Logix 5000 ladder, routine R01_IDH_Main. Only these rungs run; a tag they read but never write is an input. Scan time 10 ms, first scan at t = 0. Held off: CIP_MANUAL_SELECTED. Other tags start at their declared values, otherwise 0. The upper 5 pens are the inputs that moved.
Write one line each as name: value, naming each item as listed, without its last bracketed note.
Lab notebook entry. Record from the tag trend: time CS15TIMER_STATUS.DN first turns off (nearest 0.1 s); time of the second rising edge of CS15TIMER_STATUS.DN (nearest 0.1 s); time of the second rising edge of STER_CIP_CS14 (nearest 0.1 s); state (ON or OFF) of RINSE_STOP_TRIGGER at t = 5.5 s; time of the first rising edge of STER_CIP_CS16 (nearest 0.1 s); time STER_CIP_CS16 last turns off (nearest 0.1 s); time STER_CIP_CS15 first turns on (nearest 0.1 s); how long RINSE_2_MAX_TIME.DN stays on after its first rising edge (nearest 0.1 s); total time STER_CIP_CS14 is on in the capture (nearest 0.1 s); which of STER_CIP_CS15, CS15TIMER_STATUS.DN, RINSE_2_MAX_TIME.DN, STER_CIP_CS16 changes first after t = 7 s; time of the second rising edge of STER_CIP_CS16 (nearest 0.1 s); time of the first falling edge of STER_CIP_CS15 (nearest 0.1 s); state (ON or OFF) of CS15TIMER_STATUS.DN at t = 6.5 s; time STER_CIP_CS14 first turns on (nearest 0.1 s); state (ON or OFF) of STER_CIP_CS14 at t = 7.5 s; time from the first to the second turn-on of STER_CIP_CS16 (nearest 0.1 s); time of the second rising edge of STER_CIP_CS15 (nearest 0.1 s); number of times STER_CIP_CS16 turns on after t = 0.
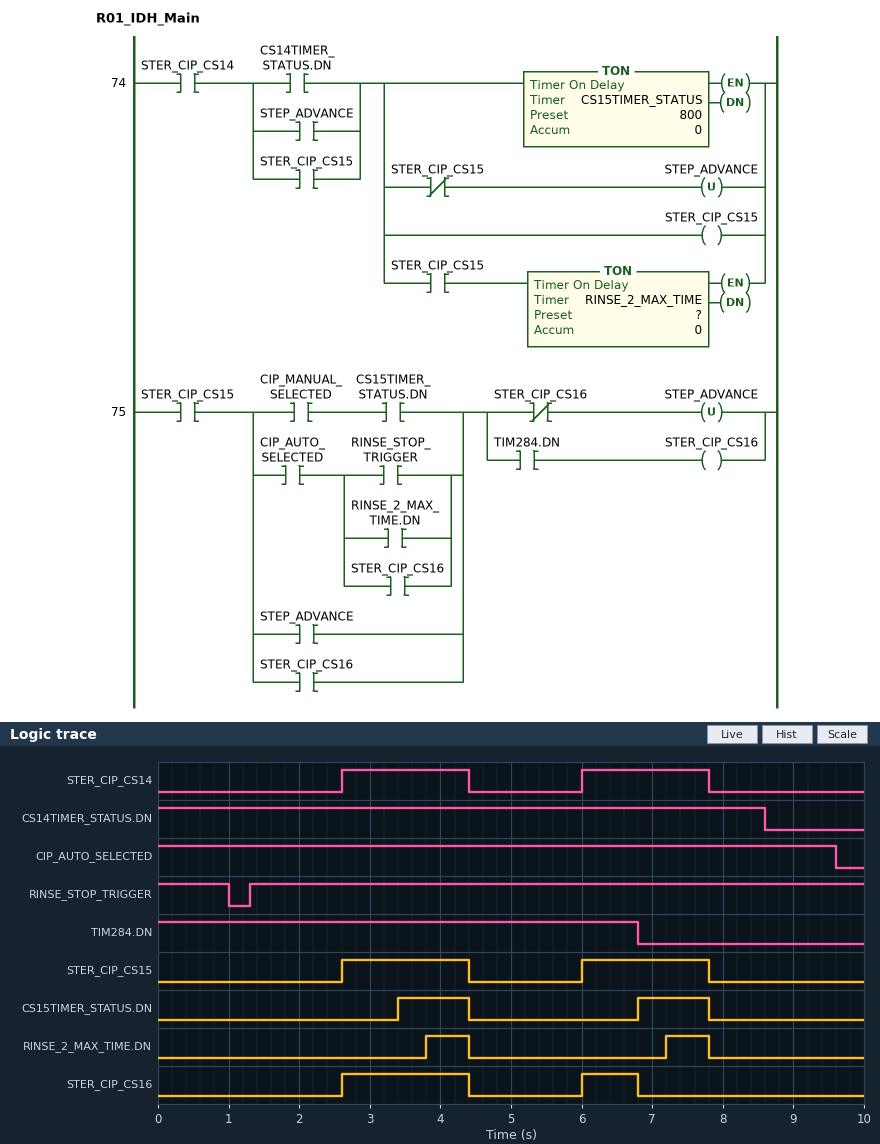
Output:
time CS15TIMER_STATUS.DN first turns off: 4.4 s
time of the second rising edge of CS15TIMER_STATUS.DN: 6.8 s
time of the second rising edge of STER_CIP_CS14: 6.0 s
state (ON or OFF) of RINSE_STOP_TRIGGER at t = 5.5 s: ON
time of the first rising edge of STER_CIP_CS16: 2.6 s
time STER_CIP_CS16 last turns off: 6.8 s
time STER_CIP_CS15 first turns on: 2.6 s
how long RINSE_2_MAX_TIME.DN stays on after its first rising edge: 0.6 s
total time STER_CIP_CS14 is on in the capture: 3.6 s
which of STER_CIP_CS15, CS15TIMER_STATUS.DN, RINSE_2_MAX_TIME.DN, STER_CIP_CS16 changes first after t = 7 s: RINSE_2_MAX_TIME.DN
time of the second rising edge of STER_CIP_CS16: 6.0 s
time of the first falling edge of STER_CIP_CS15: 4.4 s
state (ON or OFF) of CS15TIMER_STATUS.DN at t = 6.5 s: OFF
time STER_CIP_CS14 first turns on: 2.6 s
state (ON or OFF) of STER_CIP_CS14 at t = 7.5 s: ON
time from the first to the second turn-on of STER_CIP_CS16: 3.4 s
time of the second rising edge of STER_CIP_CS15: 6.0 s
number of times STER_CIP_CS16 turns on after t = 0: 2
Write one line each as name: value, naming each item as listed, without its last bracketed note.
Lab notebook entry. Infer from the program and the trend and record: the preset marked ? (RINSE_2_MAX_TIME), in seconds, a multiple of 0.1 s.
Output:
the preset marked ? (RINSE_2_MAX_TIME), in seconds, a multiple of 0.1 s: 1.2 s
